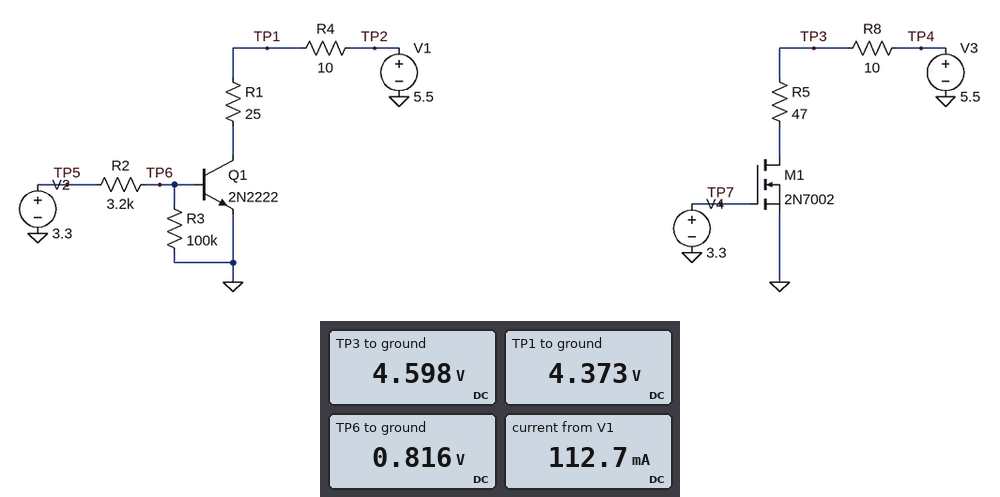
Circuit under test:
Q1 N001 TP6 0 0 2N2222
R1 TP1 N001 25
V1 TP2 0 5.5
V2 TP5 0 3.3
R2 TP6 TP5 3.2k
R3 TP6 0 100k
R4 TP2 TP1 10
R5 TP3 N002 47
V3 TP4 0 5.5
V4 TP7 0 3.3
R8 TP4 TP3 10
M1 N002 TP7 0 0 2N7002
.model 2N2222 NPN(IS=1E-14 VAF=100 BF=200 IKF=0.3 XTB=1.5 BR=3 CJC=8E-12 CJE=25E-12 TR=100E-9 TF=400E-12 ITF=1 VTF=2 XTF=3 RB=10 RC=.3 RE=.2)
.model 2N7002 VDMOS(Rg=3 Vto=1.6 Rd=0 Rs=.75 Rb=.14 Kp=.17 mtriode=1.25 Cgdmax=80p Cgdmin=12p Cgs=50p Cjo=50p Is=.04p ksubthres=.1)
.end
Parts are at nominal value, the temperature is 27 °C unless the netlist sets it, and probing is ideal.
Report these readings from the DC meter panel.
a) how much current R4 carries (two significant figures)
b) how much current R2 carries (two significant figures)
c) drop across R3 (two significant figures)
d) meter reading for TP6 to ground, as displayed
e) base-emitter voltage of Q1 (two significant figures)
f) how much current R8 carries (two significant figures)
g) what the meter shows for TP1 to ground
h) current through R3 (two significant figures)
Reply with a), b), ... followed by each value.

a) 110 mA
b) 780 µA
c) 820 mV
d) 0.816 V
e) 820 mV
f) 90 mA
g) 4.373 V
h) 8.2 µA
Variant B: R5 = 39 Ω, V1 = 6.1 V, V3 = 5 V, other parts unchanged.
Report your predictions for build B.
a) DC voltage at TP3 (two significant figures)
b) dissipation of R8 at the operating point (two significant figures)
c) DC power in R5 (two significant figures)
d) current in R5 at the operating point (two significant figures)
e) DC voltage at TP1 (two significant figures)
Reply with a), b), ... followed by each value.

a) 4.1 V
b) 89 mW
c) 350 mW
d) 94 mA
e) 5.0 V
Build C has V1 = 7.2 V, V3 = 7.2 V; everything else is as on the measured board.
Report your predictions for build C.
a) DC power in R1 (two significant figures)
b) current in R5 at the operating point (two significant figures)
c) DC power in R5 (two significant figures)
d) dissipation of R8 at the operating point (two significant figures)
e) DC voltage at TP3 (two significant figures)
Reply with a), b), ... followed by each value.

a) 330 mW
b) 120 mA
c) 650 mW
d) 140 mW
e) 6.0 V
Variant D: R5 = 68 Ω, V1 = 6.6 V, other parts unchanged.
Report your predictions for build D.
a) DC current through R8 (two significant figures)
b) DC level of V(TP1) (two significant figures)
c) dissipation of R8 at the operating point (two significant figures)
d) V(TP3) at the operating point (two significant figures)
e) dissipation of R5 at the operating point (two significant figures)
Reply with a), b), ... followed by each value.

a) 67 mA
b) 5.5 V
c) 45 mW
d) 4.8 V
e) 310 mW
